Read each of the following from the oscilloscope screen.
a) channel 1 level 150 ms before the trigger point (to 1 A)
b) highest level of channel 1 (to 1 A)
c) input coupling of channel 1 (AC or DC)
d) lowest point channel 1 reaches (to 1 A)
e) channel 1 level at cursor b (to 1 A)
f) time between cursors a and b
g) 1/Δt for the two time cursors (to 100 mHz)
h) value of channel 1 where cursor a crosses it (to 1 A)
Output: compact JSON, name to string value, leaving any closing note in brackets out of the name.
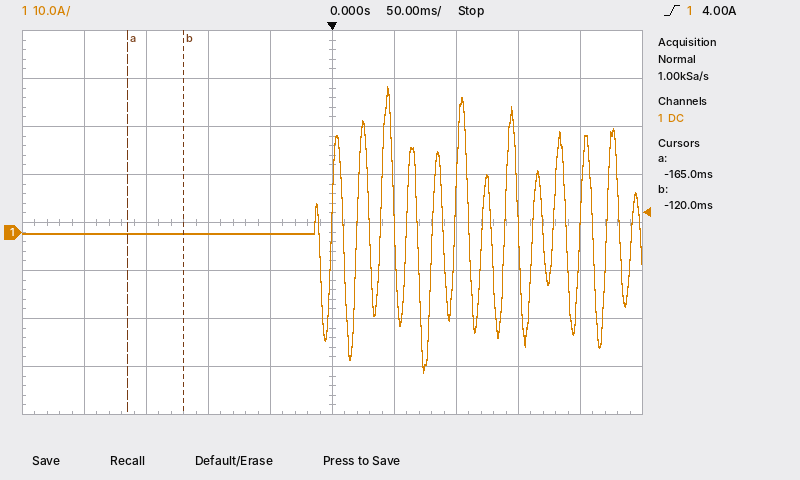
{"channel 1 level 150 ms before the trigger point": "0 A", "highest level of channel 1": "30 A", "input coupling of channel 1": "DC", "lowest point channel 1 reaches": "-29 A", "channel 1 level at cursor b": "0 A", "time between cursors a and b": "45 ms", "1/Δt for the two time cursors": "22.2 Hz", "value of channel 1 where cursor a crosses it": "0 A"}
